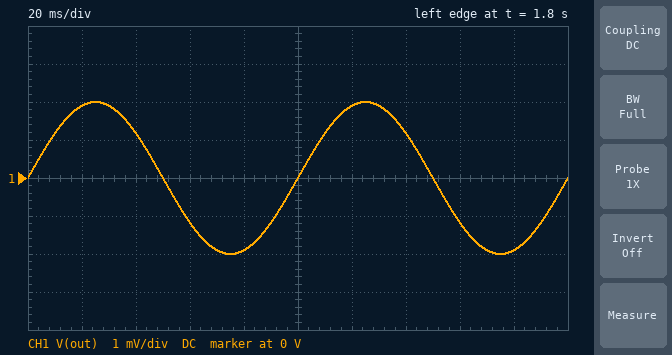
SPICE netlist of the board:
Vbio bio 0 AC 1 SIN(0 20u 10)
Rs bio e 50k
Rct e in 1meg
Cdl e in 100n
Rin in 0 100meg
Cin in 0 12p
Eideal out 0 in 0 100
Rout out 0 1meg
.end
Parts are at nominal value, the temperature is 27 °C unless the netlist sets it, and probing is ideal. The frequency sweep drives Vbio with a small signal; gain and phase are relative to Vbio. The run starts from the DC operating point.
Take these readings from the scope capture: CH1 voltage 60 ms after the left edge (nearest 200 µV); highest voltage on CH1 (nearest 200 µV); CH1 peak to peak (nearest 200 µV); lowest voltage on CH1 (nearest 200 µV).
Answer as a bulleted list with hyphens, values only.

- -1.2 mV
- 2.0 mV
- 4.0 mV
- -2.0 mV
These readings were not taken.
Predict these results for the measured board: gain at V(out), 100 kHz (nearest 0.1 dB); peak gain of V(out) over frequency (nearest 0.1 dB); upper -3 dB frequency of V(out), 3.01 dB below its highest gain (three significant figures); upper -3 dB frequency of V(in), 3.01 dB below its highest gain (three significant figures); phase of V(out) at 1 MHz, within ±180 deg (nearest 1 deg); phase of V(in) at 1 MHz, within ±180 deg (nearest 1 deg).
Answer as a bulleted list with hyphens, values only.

- 39.4 dB
- 40.0 dB
- 265 kHz
- 265 kHz
- -75 deg
- -75 deg
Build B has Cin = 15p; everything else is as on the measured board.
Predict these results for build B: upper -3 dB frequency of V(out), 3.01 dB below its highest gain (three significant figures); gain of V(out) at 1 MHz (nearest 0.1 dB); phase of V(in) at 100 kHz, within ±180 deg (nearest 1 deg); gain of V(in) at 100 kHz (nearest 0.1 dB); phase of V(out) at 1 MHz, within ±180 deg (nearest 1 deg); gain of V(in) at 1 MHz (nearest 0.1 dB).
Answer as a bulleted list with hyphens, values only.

- 212 kHz
- 26.3 dB
- -25 deg
- -0.9 dB
- -78 deg
- -13.7 dB
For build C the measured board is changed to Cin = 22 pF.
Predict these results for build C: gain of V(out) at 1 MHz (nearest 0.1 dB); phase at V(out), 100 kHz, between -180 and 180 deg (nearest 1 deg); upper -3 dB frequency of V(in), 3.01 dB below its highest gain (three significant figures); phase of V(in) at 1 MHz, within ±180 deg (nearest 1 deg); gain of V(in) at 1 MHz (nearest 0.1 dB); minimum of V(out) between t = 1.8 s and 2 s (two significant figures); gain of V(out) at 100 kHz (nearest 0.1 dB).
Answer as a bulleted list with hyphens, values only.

- 23.1 dB
- -35 deg
- 145 kHz
- -82 deg
- -16.9 dB
- -2.0 mV
- 38.3 dB
